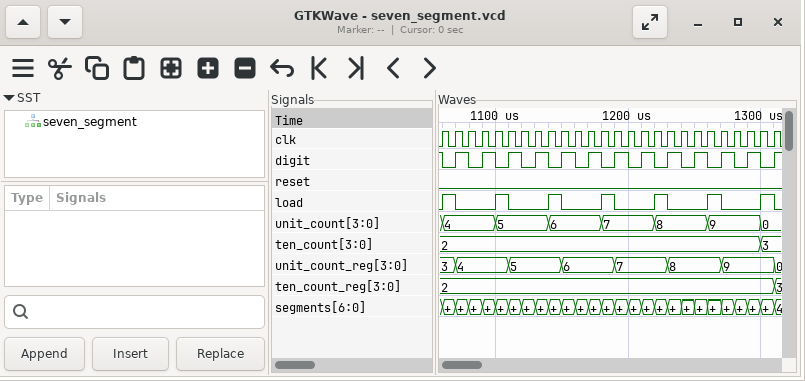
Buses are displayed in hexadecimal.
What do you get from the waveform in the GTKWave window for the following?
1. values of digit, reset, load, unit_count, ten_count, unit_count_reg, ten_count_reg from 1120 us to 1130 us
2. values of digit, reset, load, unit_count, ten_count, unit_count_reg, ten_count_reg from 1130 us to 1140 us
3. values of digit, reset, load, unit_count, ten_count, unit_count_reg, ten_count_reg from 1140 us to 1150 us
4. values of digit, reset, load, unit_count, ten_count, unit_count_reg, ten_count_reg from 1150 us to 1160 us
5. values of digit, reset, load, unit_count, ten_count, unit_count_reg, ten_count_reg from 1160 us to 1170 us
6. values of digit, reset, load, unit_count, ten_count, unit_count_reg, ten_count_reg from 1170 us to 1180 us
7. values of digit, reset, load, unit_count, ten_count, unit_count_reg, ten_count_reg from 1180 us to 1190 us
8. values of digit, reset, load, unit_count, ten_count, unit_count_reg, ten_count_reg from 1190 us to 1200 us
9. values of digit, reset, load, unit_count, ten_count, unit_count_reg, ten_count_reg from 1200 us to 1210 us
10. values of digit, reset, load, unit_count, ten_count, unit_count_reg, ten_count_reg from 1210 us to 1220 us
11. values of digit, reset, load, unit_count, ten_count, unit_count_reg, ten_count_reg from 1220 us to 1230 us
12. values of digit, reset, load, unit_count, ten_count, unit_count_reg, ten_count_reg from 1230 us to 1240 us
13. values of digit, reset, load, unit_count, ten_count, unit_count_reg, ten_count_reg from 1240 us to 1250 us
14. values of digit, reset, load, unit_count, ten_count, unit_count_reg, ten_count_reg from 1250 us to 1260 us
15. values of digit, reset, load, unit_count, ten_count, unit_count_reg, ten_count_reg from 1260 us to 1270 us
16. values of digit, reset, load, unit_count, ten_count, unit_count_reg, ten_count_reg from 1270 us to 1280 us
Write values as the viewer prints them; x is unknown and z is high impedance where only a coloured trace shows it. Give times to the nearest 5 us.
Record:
digit=0, reset=0, load=0, unit_count=5, ten_count=2, unit_count_reg=5, ten_count_reg=2
digit=1, reset=0, load=0, unit_count=5, ten_count=2, unit_count_reg=5, ten_count_reg=2
digit=0, reset=0, load=1, unit_count=6, ten_count=2, unit_count_reg=5, ten_count_reg=2
digit=1, reset=0, load=0, unit_count=6, ten_count=2, unit_count_reg=6, ten_count_reg=2
digit=0, reset=0, load=0, unit_count=6, ten_count=2, unit_count_reg=6, ten_count_reg=2
digit=1, reset=0, load=0, unit_count=6, ten_count=2, unit_count_reg=6, ten_count_reg=2
digit=0, reset=0, load=1, unit_count=7, ten_count=2, unit_count_reg=6, ten_count_reg=2
digit=1, reset=0, load=0, unit_count=7, ten_count=2, unit_count_reg=7, ten_count_reg=2
digit=0, reset=0, load=0, unit_count=7, ten_count=2, unit_count_reg=7, ten_count_reg=2
digit=1, reset=0, load=0, unit_count=7, ten_count=2, unit_count_reg=7, ten_count_reg=2
digit=0, reset=0, load=1, unit_count=8, ten_count=2, unit_count_reg=7, ten_count_reg=2
digit=1, reset=0, load=0, unit_count=8, ten_count=2, unit_count_reg=8, ten_count_reg=2
digit=0, reset=0, load=0, unit_count=8, ten_count=2, unit_count_reg=8, ten_count_reg=2
digit=1, reset=0, load=0, unit_count=8, ten_count=2, unit_count_reg=8, ten_count_reg=2
digit=0, reset=0, load=1, unit_count=9, ten_count=2, unit_count_reg=8, ten_count_reg=2
digit=1, reset=0, load=0, unit_count=9, ten_count=2, unit_count_reg=9, ten_count_reg=2
